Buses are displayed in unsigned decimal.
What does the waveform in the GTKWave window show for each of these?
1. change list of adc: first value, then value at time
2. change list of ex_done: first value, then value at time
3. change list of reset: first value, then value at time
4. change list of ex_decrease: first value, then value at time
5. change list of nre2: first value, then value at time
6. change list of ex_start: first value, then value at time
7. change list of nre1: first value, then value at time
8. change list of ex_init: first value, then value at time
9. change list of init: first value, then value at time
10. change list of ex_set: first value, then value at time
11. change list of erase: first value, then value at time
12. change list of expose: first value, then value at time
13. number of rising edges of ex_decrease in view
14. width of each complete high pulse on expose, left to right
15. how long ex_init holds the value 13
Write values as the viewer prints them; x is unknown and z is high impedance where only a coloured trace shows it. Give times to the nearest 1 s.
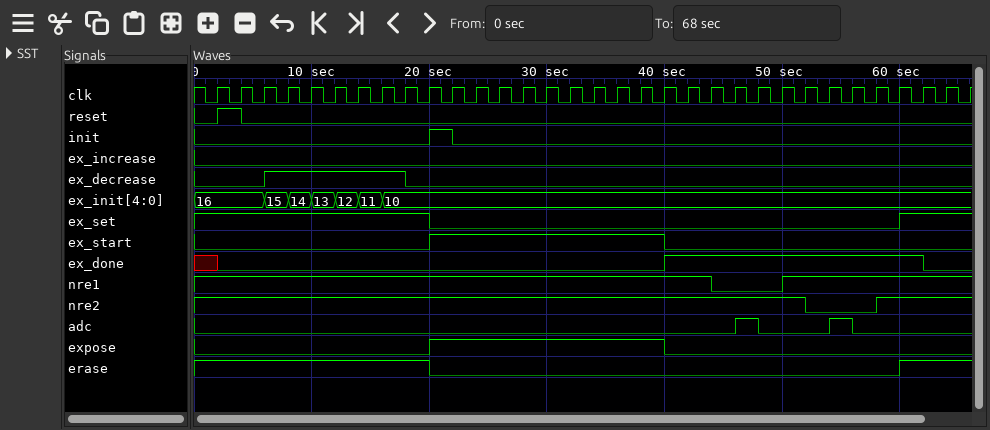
0, 1 at 46 s, 0 at 48 s, 1 at 54 s, 0 at 56 s
x, 0 at 2 s, 1 at 40 s, 0 at 62 s
0, 1 at 2 s, 0 at 4 s
0, 1 at 6 s, 0 at 18 s
1, 0 at 52 s, 1 at 58 s
0, 1 at 20 s, 0 at 40 s
1, 0 at 44 s, 1 at 50 s
16, 15 at 6 s, 14 at 8 s, 13 at 10 s, 12 at 12 s, 11 at 14 s, 10 at 16 s
0, 1 at 20 s, 0 at 22 s
1, 0 at 20 s, 1 at 60 s
1, 0 at 20 s, 1 at 60 s
0, 1 at 20 s, 0 at 40 s
1
20 s
2 s
